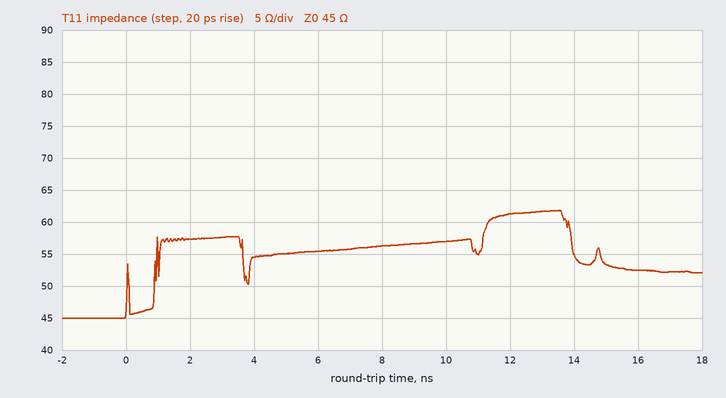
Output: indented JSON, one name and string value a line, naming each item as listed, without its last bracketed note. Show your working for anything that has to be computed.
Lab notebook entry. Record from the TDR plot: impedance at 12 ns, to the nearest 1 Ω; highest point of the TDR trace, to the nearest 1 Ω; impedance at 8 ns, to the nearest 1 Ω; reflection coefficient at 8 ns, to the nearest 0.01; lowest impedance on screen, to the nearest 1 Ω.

{
  "impedance at 12 ns, to the nearest 1 Ω": "61 Ω",
  "highest point of the TDR trace, to the nearest 1 Ω": "62 Ω",
  "impedance at 8 ns, to the nearest 1 Ω": "56 Ω",
  "reflection coefficient at 8 ns, to the nearest 0.01": "(56 − 45)/(56 + 45) ≈ +0.11",
  "lowest impedance on screen, to the nearest 1 Ω": "45 Ω"
}
